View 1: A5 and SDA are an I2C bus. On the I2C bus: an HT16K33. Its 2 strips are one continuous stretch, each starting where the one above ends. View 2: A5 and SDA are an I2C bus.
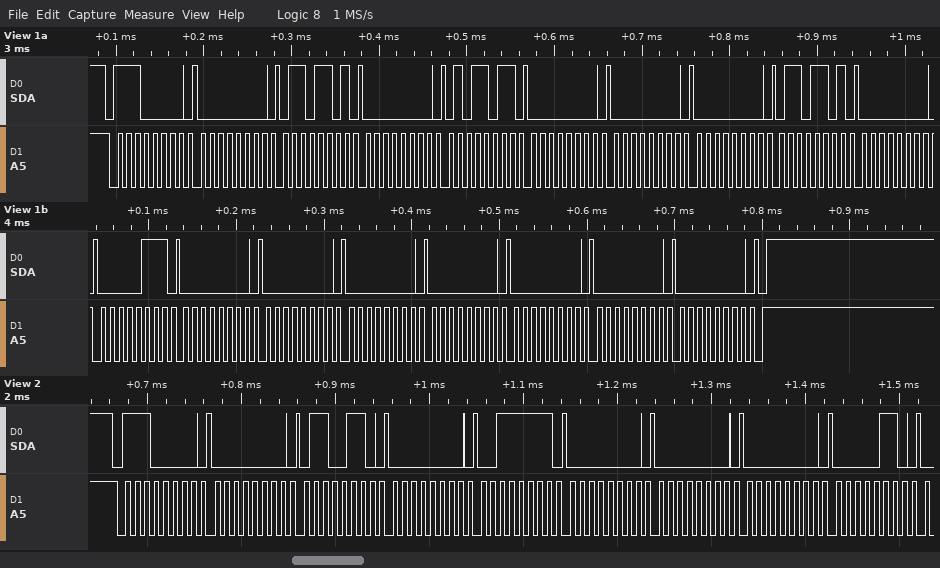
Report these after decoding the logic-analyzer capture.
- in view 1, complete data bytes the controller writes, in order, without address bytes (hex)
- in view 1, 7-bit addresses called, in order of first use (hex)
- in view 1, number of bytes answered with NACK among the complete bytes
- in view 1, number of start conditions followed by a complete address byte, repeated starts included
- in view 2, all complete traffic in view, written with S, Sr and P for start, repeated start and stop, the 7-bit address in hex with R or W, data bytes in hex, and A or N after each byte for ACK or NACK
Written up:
00 6D 00 5B 00 00 00 6D 00 07 00 00 00 00 00 00 00
0x70
0
1
S 70W A 00 A 66 A 00 A 3F A 00 A 00 A 00 A 06 A
